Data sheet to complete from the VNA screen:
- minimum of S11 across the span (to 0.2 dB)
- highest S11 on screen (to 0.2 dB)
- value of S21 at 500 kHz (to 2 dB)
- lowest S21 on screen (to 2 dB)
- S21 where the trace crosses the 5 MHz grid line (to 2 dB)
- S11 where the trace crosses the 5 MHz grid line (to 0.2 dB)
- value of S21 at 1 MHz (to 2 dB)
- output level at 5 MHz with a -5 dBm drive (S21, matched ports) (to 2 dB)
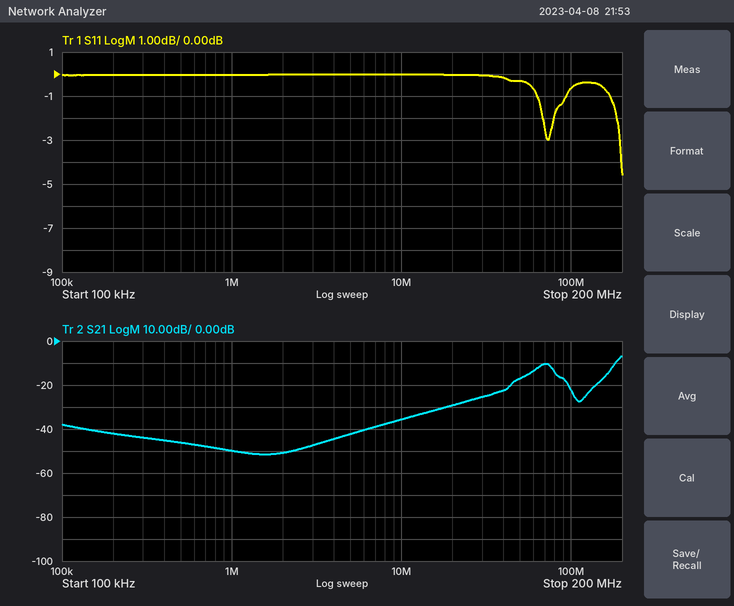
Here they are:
-4.6 dB
0.0 dB
-46 dB
-52 dB
-42 dB
0.0 dB
-50 dB
-48 dBm
